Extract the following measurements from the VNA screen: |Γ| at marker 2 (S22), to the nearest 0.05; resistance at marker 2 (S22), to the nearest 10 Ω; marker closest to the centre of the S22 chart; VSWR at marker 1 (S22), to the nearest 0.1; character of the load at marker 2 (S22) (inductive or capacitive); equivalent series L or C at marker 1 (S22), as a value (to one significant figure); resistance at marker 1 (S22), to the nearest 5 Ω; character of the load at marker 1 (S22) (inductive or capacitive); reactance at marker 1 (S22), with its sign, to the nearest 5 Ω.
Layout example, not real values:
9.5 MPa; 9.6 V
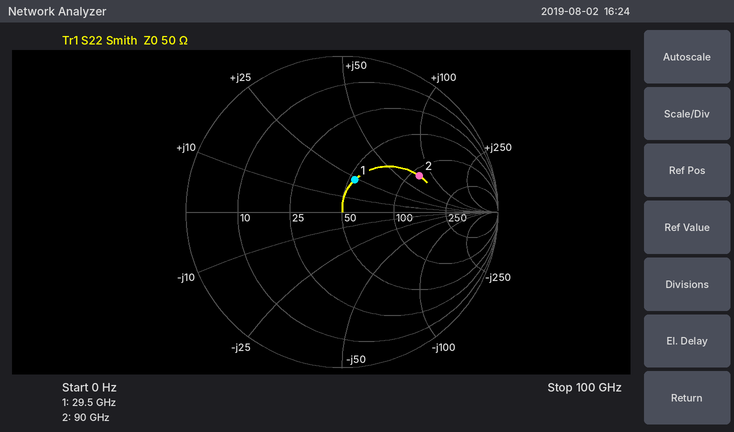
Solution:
0.55; 110 Ω; marker 1; 1.6; inductive; 100 pH; 55 Ω; inductive; +25 Ω
